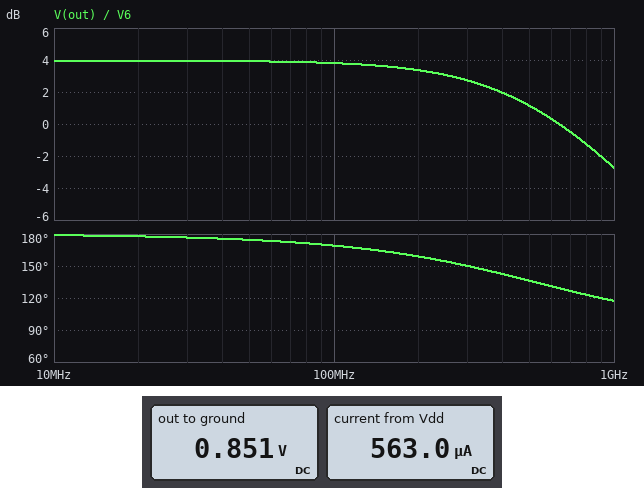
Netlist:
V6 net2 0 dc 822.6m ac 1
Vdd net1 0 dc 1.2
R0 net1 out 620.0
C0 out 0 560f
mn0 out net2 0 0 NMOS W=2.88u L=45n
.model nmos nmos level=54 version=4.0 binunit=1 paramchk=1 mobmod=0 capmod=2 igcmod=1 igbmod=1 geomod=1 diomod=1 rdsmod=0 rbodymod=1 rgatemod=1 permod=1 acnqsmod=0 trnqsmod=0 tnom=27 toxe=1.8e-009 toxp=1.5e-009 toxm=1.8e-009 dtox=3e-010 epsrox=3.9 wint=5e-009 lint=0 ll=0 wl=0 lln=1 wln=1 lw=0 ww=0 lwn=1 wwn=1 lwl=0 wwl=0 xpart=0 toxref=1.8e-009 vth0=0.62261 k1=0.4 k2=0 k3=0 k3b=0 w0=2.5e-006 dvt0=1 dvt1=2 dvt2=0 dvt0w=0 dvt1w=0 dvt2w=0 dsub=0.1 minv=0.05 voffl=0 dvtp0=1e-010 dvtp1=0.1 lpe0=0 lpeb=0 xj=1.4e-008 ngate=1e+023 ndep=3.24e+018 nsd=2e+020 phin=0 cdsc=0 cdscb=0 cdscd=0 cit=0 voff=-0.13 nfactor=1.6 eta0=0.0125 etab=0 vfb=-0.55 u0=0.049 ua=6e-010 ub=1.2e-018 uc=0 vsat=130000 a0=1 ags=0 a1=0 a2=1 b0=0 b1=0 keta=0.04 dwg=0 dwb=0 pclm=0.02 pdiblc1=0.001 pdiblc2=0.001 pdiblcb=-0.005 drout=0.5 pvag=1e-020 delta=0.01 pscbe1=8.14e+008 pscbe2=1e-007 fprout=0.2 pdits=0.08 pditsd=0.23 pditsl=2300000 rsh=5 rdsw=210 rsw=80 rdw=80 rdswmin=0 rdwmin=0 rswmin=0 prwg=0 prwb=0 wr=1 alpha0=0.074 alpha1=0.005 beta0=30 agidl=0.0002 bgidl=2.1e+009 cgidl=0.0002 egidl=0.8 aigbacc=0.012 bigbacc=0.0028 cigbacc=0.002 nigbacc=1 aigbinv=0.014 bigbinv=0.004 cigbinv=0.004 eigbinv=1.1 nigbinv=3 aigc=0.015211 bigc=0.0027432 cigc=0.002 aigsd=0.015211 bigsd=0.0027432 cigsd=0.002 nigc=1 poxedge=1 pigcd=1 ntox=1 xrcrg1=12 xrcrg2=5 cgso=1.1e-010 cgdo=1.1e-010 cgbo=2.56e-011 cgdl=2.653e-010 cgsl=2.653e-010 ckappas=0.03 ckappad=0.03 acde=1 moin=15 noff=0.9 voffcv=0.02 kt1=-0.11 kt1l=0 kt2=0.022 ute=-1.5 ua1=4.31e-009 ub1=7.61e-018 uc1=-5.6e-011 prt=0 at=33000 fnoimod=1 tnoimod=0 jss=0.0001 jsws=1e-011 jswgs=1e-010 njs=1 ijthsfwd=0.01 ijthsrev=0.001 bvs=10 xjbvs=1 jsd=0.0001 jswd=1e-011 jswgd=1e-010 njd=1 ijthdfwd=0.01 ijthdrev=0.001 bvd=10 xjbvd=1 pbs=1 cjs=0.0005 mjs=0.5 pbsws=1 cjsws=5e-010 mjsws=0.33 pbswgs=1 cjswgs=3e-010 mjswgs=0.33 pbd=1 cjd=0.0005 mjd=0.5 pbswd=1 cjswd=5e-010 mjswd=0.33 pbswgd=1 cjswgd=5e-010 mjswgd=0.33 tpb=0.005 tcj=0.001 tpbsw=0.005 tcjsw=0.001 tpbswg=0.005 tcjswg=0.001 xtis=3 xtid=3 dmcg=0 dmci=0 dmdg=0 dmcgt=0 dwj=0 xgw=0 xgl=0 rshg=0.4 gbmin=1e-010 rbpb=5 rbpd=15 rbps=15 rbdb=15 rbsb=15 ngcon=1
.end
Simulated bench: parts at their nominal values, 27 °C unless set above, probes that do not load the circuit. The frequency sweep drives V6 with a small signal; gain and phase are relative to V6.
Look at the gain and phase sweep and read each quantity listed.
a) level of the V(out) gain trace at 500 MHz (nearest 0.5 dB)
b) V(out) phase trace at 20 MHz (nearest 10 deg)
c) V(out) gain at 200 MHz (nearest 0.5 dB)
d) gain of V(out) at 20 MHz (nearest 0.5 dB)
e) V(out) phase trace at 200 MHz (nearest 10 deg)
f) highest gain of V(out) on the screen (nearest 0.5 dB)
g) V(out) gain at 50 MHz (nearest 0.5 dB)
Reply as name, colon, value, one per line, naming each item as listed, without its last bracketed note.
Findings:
level of the V(out) gain trace at 500 MHz: 1.0 dB
V(out) phase trace at 20 MHz: 180 deg
V(out) gain at 200 MHz: 3.5 dB
gain of V(out) at 20 MHz: 4.0 dB
V(out) phase trace at 200 MHz: 160 deg
highest gain of V(out) on the screen: 4.0 dB
V(out) gain at 50 MHz: 4.0 dB
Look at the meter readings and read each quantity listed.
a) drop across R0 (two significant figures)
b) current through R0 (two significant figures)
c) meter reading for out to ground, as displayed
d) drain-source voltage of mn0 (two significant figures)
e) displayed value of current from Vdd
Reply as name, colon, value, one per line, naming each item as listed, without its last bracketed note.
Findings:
drop across R0: 350 mV
current through R0: 560 µA
meter reading for out to ground, as displayed: 0.851 V
drain-source voltage of mn0: 850 mV
displayed value of current from Vdd: 563.0 µA
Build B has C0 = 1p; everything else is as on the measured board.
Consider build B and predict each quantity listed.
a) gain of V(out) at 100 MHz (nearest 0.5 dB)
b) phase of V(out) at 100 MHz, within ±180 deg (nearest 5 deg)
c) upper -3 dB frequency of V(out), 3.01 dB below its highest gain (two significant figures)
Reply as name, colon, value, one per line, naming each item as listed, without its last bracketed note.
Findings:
gain of V(out) at 100 MHz: 3.5 dB
phase of V(out) at 100 MHz, within ±180 deg: 160 deg
upper -3 dB frequency of V(out), 3.01 dB below its highest gain: 290 MHz
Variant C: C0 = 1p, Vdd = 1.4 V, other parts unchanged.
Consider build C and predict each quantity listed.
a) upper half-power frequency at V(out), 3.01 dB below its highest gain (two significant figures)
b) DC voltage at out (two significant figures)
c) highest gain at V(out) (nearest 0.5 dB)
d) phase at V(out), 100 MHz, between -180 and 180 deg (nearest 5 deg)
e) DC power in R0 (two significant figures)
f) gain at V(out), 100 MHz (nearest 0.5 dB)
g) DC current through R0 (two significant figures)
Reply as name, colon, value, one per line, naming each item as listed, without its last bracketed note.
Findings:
upper half-power frequency at V(out), 3.01 dB below its highest gain: 290 MHz
DC voltage at out: 1.0 V
highest gain at V(out): 4.0 dB
phase at V(out), 100 MHz, between -180 and 180 deg: 160 deg
DC power in R0: 230 µW
gain at V(out), 100 MHz: 3.5 dB
DC current through R0: 600 µA
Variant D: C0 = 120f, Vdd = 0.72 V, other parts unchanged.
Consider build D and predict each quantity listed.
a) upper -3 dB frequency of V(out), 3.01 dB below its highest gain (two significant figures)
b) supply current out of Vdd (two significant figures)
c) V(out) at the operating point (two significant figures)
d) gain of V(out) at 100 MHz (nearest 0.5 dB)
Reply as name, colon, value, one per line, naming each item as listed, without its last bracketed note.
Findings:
upper -3 dB frequency of V(out), 3.01 dB below its highest gain: 2.4 GHz
supply current out of Vdd: 470 µA
V(out) at the operating point: 430 mV
gain of V(out) at 100 MHz: 3.5 dB
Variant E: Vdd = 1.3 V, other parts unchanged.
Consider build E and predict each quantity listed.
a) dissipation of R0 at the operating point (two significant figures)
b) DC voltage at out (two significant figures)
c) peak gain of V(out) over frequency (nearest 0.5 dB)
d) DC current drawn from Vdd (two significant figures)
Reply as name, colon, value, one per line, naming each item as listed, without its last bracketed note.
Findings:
dissipation of R0 at the operating point: 210 µW
DC voltage at out: 940 mV
peak gain of V(out) over frequency: 4.0 dB
DC current drawn from Vdd: 580 µA
